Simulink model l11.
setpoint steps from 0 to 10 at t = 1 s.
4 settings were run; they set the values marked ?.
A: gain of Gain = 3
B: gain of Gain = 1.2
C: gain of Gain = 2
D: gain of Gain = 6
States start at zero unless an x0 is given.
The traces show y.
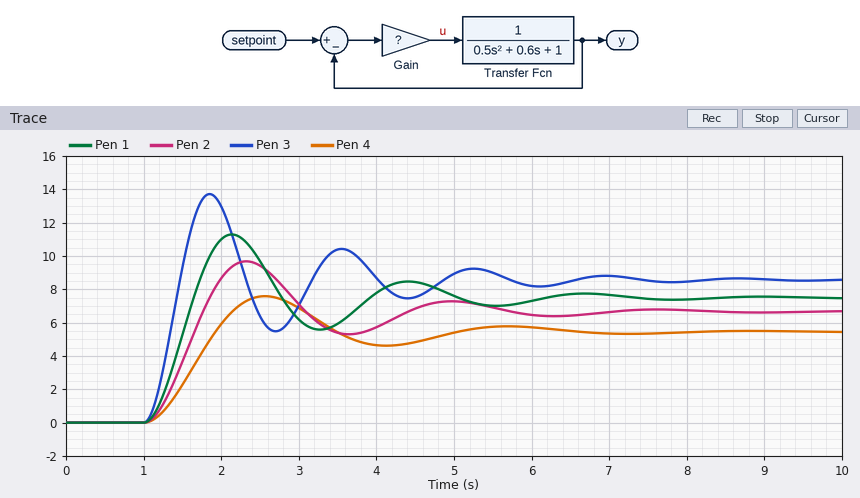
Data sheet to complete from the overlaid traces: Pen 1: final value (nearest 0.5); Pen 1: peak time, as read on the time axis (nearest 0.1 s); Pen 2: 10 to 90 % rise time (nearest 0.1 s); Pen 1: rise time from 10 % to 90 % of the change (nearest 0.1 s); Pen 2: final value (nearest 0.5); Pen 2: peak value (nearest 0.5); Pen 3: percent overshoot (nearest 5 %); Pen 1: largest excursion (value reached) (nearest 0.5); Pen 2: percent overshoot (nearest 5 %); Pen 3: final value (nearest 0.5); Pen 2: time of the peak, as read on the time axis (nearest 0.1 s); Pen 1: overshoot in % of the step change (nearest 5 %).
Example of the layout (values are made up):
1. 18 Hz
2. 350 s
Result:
1. 7.5
2. 2.1 s
3. 0.5 s
4. 0.4 s
5. 6.5
6. 9.5
7. 60 %
8. 11.5
9. 45 %
10. 8.5
11. 2.3 s
12. 50 %
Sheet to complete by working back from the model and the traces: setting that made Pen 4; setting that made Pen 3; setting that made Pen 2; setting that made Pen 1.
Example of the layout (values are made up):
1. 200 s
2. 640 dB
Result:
1. B
2. D
3. C
4. A
